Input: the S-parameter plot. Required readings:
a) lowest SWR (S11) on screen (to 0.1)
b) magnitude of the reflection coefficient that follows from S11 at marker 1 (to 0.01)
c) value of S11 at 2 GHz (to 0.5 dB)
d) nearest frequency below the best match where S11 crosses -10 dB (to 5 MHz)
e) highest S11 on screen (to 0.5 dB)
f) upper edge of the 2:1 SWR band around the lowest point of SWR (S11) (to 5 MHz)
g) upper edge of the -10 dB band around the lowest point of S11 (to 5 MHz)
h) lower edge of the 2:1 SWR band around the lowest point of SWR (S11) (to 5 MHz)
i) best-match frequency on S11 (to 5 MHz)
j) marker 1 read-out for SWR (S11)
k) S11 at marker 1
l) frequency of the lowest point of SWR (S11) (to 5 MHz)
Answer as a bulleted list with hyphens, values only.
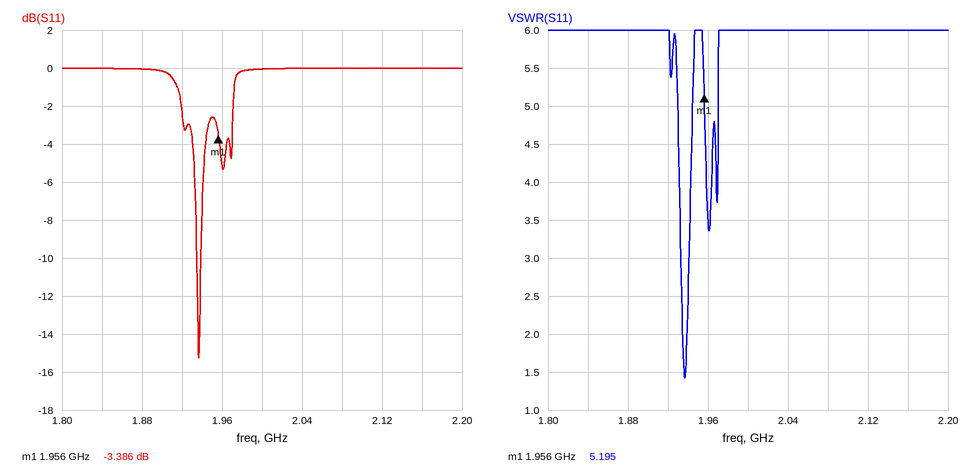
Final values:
- 1.4
- 0.68
- 0.0 dB
- 1.935 GHz
- 0.0 dB
- 1.940 GHz
- 1.940 GHz
- 1.935 GHz
- 1.935 GHz
- 5.195
- -3.386 dB
- 1.935 GHz
